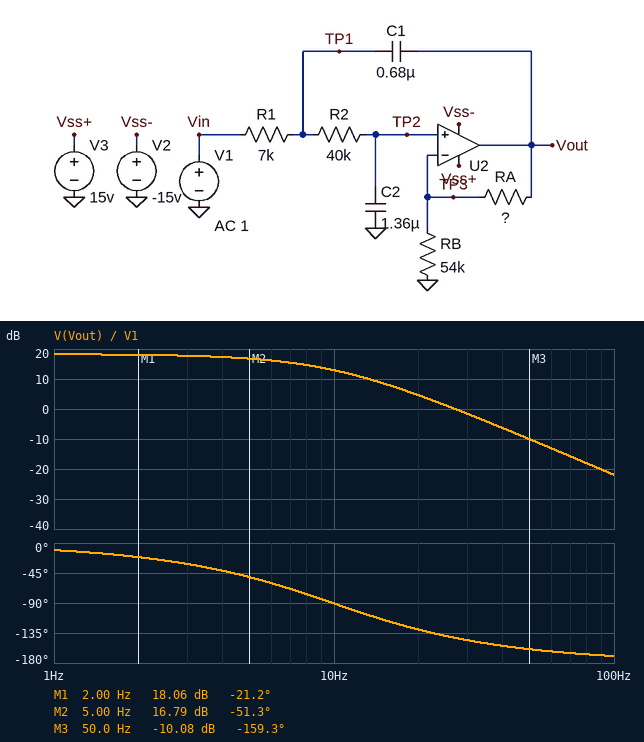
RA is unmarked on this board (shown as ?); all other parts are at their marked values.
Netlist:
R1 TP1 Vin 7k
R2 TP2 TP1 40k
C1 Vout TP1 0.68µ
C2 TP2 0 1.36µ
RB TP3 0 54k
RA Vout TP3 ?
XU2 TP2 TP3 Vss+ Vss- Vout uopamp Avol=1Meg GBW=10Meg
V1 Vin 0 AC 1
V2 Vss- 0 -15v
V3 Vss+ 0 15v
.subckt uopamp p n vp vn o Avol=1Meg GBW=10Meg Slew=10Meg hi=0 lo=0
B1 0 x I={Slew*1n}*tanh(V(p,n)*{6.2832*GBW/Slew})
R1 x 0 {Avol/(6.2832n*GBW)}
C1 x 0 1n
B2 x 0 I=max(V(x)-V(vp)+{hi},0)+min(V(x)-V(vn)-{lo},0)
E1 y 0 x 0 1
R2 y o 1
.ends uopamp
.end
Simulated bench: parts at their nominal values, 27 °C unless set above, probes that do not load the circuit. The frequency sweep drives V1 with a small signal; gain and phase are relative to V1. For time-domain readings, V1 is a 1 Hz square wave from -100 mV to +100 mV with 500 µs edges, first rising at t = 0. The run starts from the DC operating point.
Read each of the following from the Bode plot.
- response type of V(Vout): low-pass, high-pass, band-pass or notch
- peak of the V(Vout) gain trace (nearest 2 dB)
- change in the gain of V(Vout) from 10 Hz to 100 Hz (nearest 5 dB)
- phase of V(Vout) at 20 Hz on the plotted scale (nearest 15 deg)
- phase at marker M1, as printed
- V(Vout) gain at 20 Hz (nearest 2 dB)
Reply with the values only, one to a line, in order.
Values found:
low-pass
18 dB
-35 dB
-135 deg
-21.2 deg
4 dB
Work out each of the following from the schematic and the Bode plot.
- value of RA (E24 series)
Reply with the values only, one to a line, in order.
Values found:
390 kΩ
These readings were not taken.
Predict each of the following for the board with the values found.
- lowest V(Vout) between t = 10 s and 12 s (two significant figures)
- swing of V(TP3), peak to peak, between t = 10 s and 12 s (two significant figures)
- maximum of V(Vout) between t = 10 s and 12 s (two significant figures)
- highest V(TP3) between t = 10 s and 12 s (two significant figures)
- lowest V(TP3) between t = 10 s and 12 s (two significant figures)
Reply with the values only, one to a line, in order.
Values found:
-820 mV
200 mV
820 mV
100 mV
-100 mV
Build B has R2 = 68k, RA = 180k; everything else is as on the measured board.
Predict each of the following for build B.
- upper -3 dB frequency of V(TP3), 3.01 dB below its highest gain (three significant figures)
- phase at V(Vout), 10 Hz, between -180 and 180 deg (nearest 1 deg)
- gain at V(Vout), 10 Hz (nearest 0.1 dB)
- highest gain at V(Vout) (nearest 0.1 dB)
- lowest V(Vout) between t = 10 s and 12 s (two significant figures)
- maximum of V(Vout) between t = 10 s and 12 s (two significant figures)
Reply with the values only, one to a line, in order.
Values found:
1.96 Hz
-98 deg
-2.0 dB
12.7 dB
-430 mV
430 mV
